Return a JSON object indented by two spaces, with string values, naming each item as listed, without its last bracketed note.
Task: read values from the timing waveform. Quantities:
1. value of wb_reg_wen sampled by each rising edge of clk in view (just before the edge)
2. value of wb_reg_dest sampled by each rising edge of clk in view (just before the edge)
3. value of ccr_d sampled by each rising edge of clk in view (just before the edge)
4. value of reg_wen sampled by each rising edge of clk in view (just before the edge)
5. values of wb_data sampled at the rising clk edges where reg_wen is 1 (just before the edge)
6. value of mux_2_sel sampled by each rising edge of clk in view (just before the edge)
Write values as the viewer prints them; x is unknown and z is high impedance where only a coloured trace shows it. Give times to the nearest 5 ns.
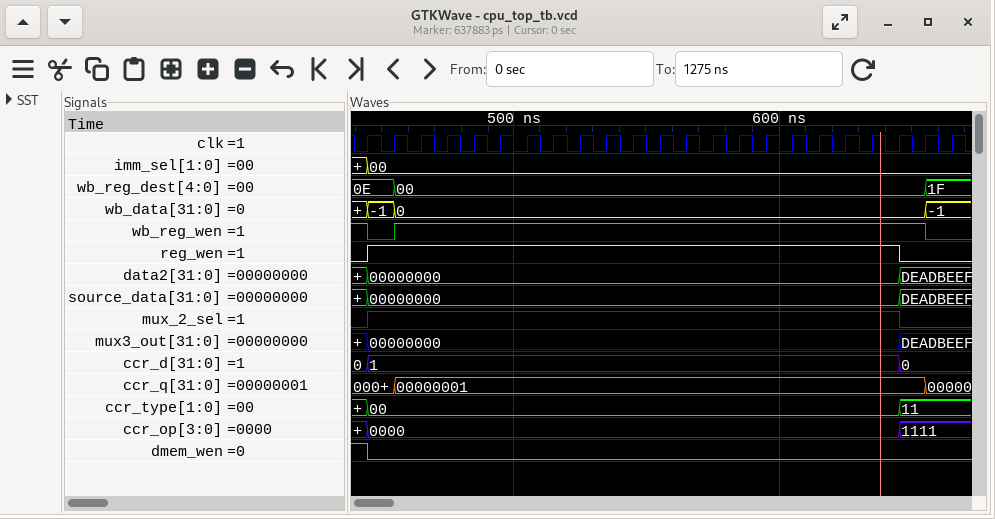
{
  "value of wb_reg_wen sampled by each rising edge of clk in view": "1 0 1 1 1 1 1 1 1 1 1 1 1 1 1 1 1 1 1 1 1 1 0",
  "value of wb_reg_dest sampled by each rising edge of clk in view": "0E, 0E, 00, 00, 00, 00, 00, 00, 00, 00, 00, 00, 00, 00, 00, 00, 00, 00, 00, 00, 00, 00, 1F",
  "value of ccr_d sampled by each rising edge of clk in view": "0, 1, 1, 1, 1, 1, 1, 1, 1, 1, 1, 1, 1, 1, 1, 1, 1, 1, 1, 1, 1, 0, 0",
  "value of reg_wen sampled by each rising edge of clk in view": "0 1 1 1 1 1 1 1 1 1 1 1 1 1 1 1 1 1 1 1 1 0 0",
  "values of wb_data sampled at the rising clk edges where reg_wen is 1": "-1, 0, 0, 0, 0, 0, 0, 0, 0, 0, 0, 0, 0, 0, 0, 0, 0, 0, 0, 0",
  "value of mux_2_sel sampled by each rising edge of clk in view": "0 1 1 1 1 1 1 1 1 1 1 1 1 1 1 1 1 1 1 1 1 0 0"
}
